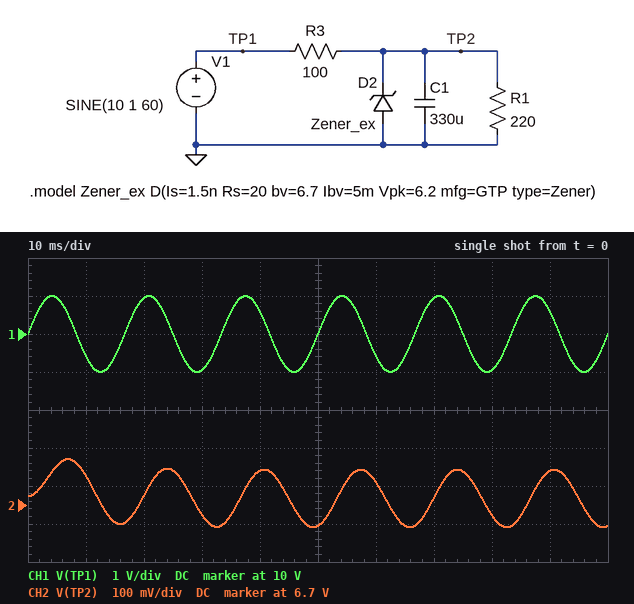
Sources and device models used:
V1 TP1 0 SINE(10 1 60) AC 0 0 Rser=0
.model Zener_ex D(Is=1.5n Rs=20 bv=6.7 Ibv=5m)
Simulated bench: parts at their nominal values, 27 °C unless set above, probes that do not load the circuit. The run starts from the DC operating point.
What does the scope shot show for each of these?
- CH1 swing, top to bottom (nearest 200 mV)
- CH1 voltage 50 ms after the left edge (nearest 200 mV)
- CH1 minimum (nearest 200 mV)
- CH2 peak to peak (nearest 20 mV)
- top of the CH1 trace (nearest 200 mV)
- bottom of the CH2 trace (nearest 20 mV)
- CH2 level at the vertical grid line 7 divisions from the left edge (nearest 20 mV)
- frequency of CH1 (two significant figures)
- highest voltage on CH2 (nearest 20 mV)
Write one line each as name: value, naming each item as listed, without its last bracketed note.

CH1 swing, top to bottom: 2.0 V
CH1 voltage 50 ms after the left edge: 10.0 V
CH1 minimum: 9.0 V
CH2 peak to peak: 180 mV
top of the CH1 trace: 11.0 V
bottom of the CH2 trace: 6.64 V
CH2 level at the vertical grid line 7 divisions from the left edge: 6.72 V
frequency of CH1: 60 Hz
highest voltage on CH2: 6.82 V
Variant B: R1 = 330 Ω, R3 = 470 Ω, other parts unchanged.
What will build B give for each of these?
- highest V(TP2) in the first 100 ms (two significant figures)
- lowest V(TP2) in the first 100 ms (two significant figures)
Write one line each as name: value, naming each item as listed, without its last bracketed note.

highest V(TP2) in the first 100 ms: 4.2 V
lowest V(TP2) in the first 100 ms: 4.1 V
